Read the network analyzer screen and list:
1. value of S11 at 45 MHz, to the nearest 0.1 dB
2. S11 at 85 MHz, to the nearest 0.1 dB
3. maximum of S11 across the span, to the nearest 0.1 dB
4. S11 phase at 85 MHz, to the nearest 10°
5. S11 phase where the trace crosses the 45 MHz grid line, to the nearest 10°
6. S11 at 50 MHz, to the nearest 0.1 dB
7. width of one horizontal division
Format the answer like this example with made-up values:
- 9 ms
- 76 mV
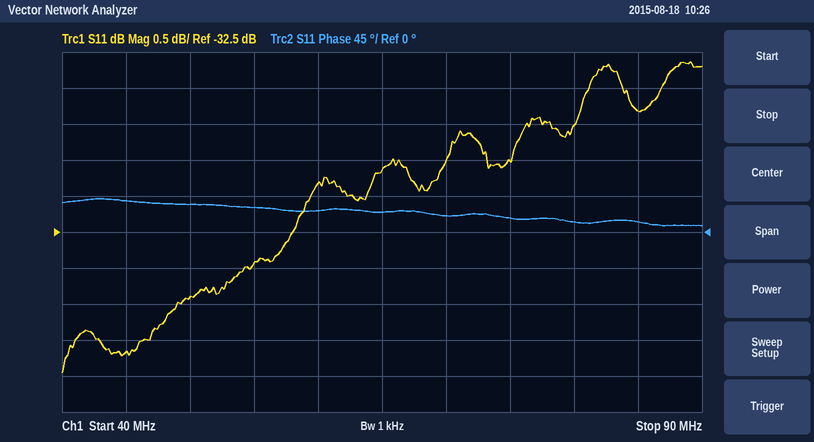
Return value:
- -34.2 dB
- -30.8 dB
- -30.1 dB
- 10°
- 40°
- -33.4 dB
- 5 MHz
